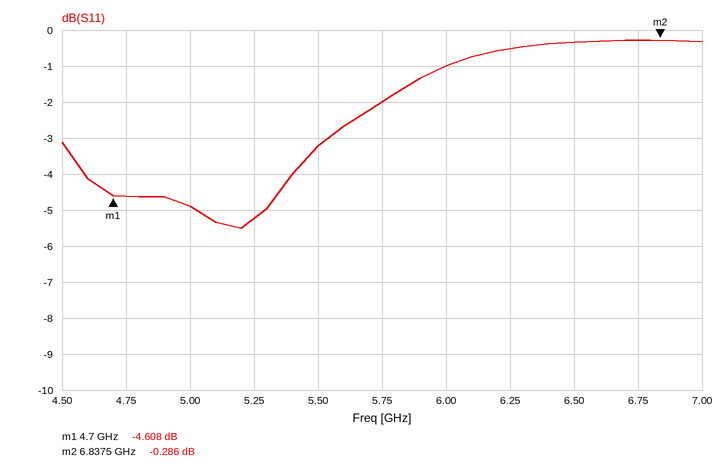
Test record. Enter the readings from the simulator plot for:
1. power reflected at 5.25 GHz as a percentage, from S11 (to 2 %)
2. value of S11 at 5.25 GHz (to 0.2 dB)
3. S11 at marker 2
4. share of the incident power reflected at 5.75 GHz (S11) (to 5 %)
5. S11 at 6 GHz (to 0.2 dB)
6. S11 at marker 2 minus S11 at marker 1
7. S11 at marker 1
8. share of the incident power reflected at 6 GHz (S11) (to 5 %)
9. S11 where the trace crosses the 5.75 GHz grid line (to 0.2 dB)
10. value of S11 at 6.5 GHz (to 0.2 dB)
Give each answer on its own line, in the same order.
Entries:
30 %
-5.2 dB
-0.286 dB
65 %
-1.0 dB
4.322 dB
-4.608 dB
80 %
-2.0 dB
-0.4 dB
